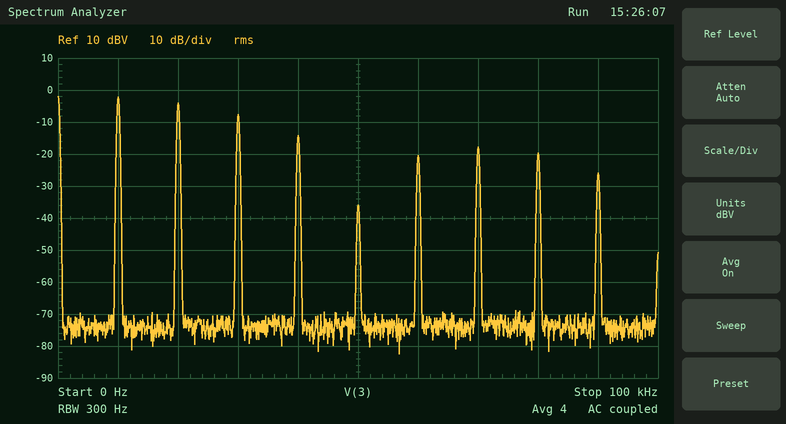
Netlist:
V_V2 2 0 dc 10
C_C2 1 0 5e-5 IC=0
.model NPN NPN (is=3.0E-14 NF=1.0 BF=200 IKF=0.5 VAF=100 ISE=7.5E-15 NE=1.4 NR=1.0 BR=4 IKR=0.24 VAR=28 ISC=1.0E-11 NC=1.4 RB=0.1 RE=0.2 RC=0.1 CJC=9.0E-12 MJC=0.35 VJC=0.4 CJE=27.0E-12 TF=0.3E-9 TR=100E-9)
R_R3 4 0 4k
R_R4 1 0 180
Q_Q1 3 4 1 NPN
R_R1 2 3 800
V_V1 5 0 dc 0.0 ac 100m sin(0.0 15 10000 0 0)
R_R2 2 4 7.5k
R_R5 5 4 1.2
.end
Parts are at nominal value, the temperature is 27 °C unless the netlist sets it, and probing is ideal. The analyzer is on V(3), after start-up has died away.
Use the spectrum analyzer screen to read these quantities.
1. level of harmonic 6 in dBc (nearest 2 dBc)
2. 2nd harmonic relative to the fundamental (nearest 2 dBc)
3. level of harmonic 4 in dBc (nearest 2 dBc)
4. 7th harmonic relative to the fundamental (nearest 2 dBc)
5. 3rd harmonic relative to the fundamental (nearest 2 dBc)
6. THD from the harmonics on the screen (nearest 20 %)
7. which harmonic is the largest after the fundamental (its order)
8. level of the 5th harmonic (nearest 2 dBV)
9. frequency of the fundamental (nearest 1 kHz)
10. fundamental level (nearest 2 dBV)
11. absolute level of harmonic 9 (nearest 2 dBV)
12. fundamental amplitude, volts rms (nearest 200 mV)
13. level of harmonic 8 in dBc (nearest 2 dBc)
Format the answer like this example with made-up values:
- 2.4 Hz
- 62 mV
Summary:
- -18 dBc
- -2 dBc
- -12 dBc
- -16 dBc
- -6 dBc
- 100 %
- 2
- -36 dBV
- 10 kHz
- -2 dBV
- -26 dBV
- 800 mV
- -18 dBc
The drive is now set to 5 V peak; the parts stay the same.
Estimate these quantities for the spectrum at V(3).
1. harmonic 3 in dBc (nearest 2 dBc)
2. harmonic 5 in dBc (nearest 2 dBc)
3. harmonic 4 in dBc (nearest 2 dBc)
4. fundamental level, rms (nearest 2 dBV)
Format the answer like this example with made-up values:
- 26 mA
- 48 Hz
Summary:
- -2 dBc
- -10 dBc
- -6 dBc
- 2 dBV
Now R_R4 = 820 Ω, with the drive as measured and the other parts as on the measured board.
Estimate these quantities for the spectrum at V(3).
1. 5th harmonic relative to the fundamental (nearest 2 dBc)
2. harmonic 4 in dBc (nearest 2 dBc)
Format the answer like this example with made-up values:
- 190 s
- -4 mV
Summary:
- -22 dBc
- -10 dBc
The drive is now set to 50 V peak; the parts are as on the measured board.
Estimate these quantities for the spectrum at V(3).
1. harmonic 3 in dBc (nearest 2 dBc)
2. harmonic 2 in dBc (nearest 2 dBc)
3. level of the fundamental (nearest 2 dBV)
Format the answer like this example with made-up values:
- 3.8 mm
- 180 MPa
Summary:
- -22 dBc
- -6 dBc
- 22 dBV
